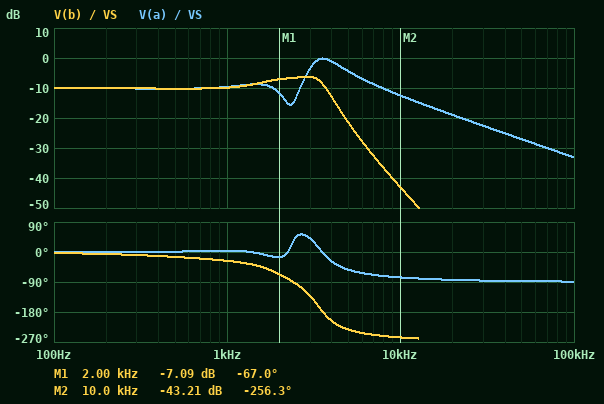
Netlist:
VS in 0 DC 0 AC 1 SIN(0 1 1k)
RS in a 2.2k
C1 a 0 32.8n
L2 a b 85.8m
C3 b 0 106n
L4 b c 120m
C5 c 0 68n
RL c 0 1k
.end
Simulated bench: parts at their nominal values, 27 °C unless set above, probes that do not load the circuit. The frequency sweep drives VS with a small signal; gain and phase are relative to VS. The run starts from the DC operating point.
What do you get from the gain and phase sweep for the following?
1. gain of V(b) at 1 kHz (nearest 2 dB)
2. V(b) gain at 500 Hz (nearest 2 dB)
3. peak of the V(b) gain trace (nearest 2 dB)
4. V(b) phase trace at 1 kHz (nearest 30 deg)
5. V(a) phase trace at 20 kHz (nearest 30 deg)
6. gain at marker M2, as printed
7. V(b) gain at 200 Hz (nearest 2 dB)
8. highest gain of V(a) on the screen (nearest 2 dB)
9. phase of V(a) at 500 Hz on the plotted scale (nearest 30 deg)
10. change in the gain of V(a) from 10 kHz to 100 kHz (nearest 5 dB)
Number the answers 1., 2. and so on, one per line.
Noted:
1. -10 dB
2. -10 dB
3. -6 dB
4. -30 deg
5. -90 deg
6. -43.21 dB
7. -10 dB
8. 0 dB
9. 0 deg
10. -20 dB
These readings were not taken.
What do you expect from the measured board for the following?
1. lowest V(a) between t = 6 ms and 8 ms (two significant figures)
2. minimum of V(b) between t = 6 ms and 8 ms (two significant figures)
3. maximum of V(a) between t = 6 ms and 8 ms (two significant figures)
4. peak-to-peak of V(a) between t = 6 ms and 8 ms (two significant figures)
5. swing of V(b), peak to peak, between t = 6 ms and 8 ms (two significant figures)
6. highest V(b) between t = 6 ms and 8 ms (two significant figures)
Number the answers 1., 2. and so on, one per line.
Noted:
1. -330 mV
2. -320 mV
3. 330 mV
4. 660 mV
5. 640 mV
6. 320 mV
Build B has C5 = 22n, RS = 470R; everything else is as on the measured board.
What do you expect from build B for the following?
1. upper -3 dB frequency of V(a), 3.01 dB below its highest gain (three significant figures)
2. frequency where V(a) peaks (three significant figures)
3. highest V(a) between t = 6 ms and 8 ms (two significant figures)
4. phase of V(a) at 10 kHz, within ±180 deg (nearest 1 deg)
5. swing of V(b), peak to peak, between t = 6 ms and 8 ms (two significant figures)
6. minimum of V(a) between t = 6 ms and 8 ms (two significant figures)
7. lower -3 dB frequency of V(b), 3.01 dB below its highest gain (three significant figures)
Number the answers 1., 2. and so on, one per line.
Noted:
1. 11.3 kHz
2. 3.72 kHz
3. 730 mV
4. -41 deg
5. 1.5 V
6. -730 mV
7. 1.38 kHz
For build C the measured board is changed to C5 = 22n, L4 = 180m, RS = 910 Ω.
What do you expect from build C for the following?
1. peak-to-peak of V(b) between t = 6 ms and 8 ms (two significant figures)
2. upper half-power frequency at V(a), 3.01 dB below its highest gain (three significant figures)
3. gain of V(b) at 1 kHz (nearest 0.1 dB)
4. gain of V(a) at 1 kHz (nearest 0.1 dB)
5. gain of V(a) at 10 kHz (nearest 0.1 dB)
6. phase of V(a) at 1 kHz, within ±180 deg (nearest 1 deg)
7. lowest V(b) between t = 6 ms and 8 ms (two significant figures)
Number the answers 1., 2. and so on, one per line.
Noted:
1. 1.4 V
2. 6.81 kHz
3. -3.2 dB
4. -3.6 dB
5. -5.9 dB
6. -7 deg
7. -690 mV
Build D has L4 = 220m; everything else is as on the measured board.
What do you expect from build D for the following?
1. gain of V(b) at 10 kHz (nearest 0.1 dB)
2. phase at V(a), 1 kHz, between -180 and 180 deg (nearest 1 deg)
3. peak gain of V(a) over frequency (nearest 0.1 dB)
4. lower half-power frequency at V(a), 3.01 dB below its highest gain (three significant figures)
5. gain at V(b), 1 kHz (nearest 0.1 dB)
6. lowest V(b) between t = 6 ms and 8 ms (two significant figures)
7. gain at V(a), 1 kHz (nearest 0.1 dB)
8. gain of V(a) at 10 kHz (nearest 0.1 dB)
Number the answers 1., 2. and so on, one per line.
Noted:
1. -43.3 dB
2. -10 deg
3. 0 dB
4. 2.90 kHz
5. -6.4 dB
6. -480 mV
7. -6.5 dB
8. -12.5 dB
